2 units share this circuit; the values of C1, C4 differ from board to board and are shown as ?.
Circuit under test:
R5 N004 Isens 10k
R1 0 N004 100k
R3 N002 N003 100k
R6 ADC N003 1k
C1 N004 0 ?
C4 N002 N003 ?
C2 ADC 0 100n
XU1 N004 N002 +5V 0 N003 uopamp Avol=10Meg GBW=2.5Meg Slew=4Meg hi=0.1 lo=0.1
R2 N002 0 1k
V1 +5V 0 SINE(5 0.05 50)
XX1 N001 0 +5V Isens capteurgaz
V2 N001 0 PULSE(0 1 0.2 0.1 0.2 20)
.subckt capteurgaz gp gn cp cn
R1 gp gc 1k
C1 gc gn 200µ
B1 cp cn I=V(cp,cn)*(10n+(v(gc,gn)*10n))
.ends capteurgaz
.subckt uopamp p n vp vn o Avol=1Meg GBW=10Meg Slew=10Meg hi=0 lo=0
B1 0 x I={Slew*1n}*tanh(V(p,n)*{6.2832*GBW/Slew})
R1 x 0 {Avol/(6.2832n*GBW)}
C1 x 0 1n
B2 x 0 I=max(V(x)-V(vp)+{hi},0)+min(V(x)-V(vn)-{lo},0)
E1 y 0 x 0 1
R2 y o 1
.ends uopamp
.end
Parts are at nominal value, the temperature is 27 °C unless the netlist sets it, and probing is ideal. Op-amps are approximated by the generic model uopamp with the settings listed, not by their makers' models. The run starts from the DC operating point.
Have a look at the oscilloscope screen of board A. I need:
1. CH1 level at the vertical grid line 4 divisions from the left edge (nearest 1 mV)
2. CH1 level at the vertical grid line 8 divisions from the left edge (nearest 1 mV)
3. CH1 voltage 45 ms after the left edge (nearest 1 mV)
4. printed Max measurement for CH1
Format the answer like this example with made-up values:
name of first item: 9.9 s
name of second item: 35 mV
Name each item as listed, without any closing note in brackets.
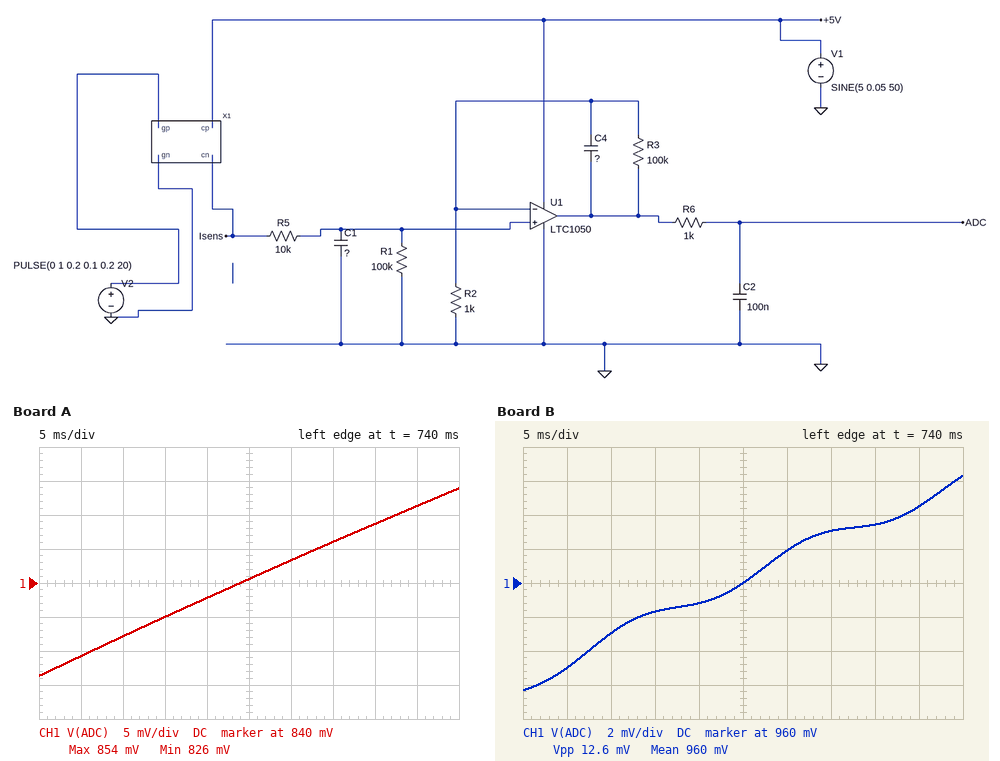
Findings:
CH1 level at the vertical grid line 4 divisions from the left edge: 838 mV
CH1 level at the vertical grid line 8 divisions from the left edge: 849 mV
CH1 voltage 45 ms after the left edge: 851 mV
printed Max measurement for CH1: 854 mV
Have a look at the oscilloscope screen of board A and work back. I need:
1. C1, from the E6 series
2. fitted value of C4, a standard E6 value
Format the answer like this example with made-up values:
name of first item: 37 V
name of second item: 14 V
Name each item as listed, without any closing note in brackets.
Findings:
C1, from the E6 series: 330 nF
fitted value of C4, a standard E6 value: 2.2 µF
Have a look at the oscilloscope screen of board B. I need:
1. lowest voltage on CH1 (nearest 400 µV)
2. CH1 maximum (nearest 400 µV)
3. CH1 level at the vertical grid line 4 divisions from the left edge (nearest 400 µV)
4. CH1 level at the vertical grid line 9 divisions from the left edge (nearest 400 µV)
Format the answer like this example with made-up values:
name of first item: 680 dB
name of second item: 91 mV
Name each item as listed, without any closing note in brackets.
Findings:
lowest voltage on CH1: 953.6 mV
CH1 maximum: 966.4 mV
CH1 level at the vertical grid line 4 divisions from the left edge: 958.8 mV
CH1 level at the vertical grid line 9 divisions from the left edge: 964.4 mV
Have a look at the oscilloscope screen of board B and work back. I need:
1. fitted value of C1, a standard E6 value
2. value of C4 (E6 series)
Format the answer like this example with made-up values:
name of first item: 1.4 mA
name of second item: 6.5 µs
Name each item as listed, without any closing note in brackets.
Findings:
fitted value of C1, a standard E6 value: 47 nF
value of C4: 330 nF
